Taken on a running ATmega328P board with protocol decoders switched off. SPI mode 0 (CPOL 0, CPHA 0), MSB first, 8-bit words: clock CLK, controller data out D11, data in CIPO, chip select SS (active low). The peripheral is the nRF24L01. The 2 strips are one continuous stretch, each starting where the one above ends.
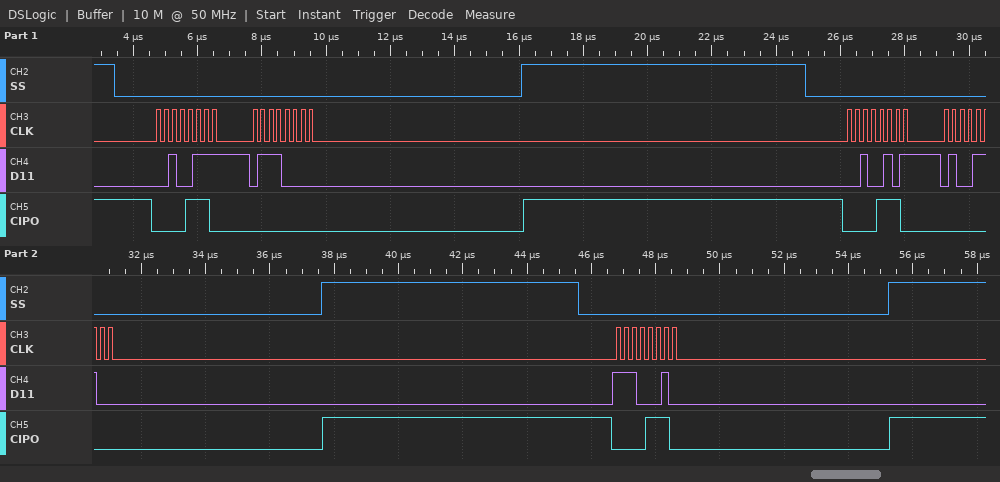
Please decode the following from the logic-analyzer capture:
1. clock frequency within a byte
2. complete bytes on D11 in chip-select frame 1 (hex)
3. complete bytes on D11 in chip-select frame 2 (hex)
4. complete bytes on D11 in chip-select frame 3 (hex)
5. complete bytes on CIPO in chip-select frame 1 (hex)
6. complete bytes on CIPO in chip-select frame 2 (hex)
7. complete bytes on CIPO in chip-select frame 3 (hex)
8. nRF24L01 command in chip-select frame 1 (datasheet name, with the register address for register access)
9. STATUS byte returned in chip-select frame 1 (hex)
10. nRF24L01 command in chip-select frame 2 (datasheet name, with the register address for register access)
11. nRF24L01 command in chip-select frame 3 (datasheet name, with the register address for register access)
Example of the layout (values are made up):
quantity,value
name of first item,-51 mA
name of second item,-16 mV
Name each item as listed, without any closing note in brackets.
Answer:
quantity,value
clock frequency within a byte,4 MHz
complete bytes on D11 in chip-select frame 1,27 70
complete bytes on D11 in chip-select frame 2,25 4C
complete bytes on D11 in chip-select frame 3,E2
complete bytes on CIPO in chip-select frame 1,0E 00
complete bytes on CIPO in chip-select frame 2,0E 00
complete bytes on CIPO in chip-select frame 3,0E
nRF24L01 command in chip-select frame 1,W_REGISTER 0x07
STATUS byte returned in chip-select frame 1,0x0E
nRF24L01 command in chip-select frame 2,W_REGISTER 0x05
nRF24L01 command in chip-select frame 3,FLUSH_RX
